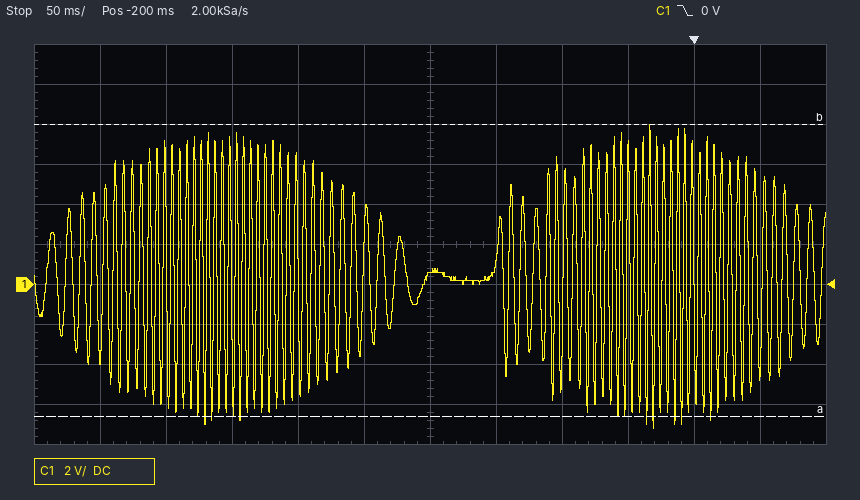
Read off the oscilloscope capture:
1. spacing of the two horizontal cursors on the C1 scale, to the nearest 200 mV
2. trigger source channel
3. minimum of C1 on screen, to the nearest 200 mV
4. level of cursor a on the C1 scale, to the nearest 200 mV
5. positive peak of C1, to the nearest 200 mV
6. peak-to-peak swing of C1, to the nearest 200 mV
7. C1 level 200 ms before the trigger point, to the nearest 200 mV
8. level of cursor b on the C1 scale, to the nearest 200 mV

14.6 V
C1
-7.2 V
-6.6 V
8.0 V
15.2 V
600 mV
8.0 V
